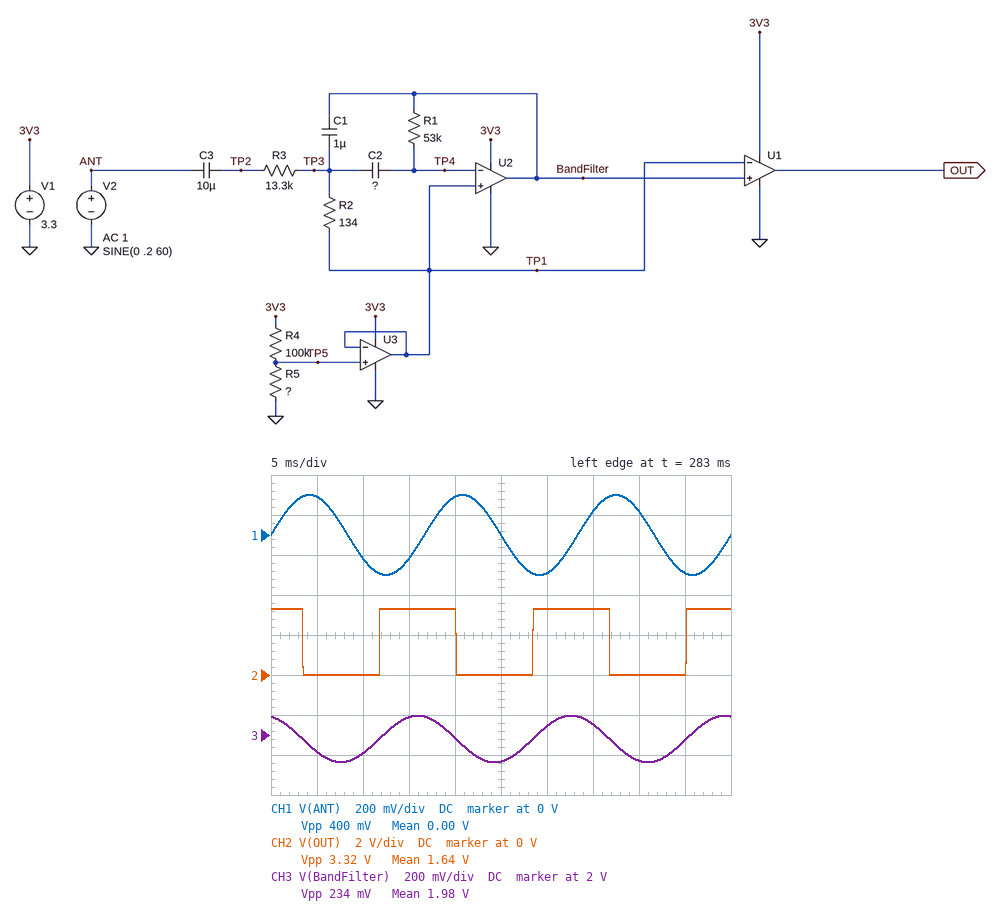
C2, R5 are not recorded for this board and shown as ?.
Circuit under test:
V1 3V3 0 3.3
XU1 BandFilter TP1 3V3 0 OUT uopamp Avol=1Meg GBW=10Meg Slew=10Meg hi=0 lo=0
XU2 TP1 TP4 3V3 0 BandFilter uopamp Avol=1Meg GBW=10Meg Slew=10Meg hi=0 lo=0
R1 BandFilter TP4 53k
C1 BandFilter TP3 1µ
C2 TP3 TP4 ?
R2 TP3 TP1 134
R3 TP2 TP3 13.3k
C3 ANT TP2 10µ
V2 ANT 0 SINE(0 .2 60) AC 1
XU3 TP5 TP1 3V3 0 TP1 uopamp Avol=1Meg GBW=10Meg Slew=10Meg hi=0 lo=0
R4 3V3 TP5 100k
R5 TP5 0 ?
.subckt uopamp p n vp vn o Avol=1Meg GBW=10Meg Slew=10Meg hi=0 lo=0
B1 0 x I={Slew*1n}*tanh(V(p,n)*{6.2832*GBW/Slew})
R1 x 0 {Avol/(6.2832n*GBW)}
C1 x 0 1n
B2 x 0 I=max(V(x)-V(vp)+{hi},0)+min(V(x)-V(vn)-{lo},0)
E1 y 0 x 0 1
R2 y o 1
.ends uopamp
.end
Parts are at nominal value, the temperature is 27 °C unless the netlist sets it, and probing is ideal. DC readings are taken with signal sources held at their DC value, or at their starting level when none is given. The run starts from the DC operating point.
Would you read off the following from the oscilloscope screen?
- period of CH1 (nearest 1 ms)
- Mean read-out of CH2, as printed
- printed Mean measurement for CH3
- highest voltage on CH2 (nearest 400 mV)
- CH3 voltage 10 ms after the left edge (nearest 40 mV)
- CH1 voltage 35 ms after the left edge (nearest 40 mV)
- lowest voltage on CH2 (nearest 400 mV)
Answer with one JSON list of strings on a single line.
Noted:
["17 ms", "1.64 V", "1.98 V", "3.2 V", "1.92 V", "120 mV", "0 V"]
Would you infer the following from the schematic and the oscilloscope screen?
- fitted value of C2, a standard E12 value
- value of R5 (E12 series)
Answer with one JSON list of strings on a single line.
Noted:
["1.5 µF", "150 kΩ"]
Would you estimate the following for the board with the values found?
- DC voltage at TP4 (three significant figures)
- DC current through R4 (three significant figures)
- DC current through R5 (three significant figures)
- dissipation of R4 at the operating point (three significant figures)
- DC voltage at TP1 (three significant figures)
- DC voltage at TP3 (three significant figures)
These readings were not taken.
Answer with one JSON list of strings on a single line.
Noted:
["1.98 V", "13.2 µA", "13.2 µA", "17.4 µW", "1.98 V", "1.98 V"]
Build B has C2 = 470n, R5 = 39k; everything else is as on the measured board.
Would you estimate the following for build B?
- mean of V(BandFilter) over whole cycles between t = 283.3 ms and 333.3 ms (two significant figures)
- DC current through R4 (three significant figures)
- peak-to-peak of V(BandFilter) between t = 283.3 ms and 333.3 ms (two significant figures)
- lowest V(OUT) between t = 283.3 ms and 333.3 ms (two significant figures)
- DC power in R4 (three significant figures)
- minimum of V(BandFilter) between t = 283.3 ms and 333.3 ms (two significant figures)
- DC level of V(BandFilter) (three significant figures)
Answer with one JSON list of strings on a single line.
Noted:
["930 mV", "23.7 µA", "70 mV", "-2.2 mV", "56.4 µW", "890 mV", "926 mV"]
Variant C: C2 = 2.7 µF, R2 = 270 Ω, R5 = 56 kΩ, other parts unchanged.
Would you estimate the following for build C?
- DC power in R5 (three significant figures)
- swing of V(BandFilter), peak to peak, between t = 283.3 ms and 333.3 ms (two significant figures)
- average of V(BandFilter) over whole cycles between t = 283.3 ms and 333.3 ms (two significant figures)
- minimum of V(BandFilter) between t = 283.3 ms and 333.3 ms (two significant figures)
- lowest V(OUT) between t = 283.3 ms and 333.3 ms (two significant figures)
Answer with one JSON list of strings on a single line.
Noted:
["25.1 µW", "99 mV", "1.2 V", "1.1 V", "-3.0 mV"]
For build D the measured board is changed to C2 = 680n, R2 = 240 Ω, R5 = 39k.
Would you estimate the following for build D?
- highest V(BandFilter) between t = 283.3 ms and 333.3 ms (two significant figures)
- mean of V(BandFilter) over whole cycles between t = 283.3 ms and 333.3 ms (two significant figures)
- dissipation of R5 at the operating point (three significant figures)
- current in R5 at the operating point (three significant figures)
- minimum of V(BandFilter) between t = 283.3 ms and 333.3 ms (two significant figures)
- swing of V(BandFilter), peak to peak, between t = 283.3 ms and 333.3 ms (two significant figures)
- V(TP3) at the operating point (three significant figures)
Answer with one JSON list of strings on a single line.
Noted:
["1.1 V", "930 mV", "22.0 µW", "23.7 µA", "740 mV", "380 mV", "926 mV"]
